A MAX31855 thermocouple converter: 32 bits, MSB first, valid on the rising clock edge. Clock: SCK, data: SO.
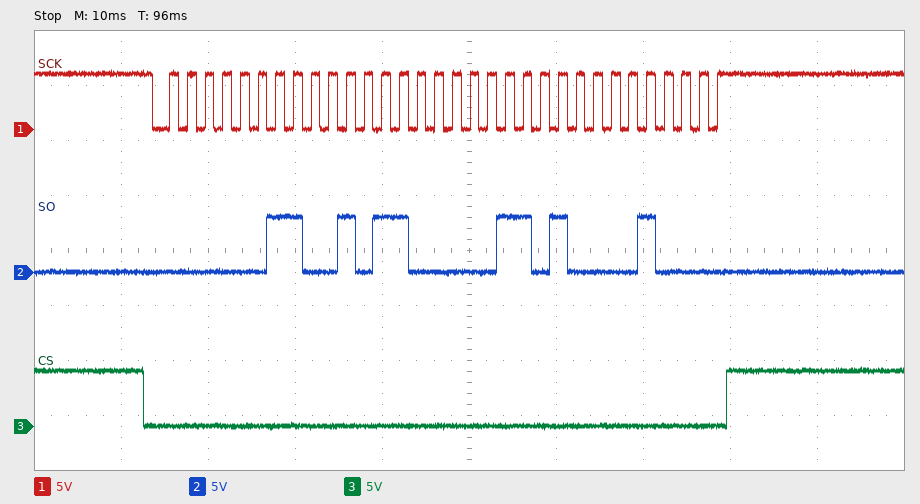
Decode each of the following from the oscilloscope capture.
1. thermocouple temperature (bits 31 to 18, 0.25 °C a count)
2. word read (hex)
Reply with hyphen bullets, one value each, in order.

- 50.75 °C
- 0x032C1A10
